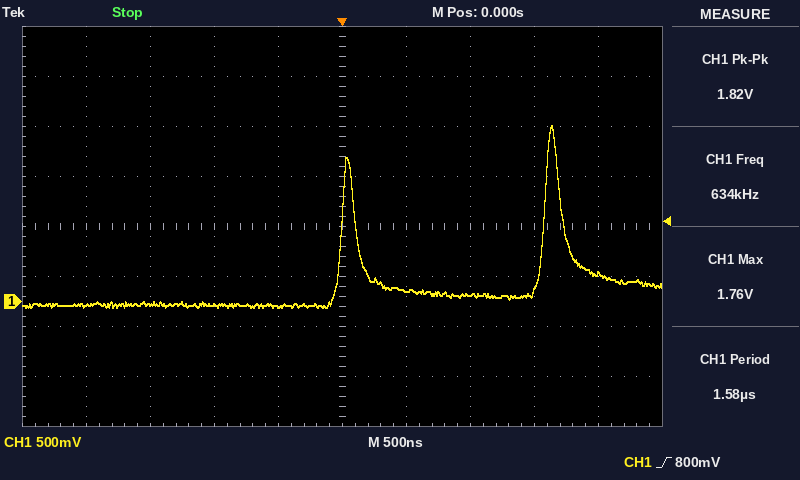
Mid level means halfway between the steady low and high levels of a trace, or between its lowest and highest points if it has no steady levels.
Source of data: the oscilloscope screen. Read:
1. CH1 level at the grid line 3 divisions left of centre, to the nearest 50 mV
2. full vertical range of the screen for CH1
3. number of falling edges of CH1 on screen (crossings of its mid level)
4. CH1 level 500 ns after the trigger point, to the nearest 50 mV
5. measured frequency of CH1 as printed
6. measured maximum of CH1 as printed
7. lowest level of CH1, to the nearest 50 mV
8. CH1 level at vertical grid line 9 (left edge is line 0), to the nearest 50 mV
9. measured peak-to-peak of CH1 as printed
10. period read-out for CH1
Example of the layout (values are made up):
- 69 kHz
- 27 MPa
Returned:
- -50 mV
- 4 V
- 2
- 100 mV
- 634 kHz
- 1.76 V
- -50 mV
- 300 mV
- 1.82 V
- 1.58 µs
